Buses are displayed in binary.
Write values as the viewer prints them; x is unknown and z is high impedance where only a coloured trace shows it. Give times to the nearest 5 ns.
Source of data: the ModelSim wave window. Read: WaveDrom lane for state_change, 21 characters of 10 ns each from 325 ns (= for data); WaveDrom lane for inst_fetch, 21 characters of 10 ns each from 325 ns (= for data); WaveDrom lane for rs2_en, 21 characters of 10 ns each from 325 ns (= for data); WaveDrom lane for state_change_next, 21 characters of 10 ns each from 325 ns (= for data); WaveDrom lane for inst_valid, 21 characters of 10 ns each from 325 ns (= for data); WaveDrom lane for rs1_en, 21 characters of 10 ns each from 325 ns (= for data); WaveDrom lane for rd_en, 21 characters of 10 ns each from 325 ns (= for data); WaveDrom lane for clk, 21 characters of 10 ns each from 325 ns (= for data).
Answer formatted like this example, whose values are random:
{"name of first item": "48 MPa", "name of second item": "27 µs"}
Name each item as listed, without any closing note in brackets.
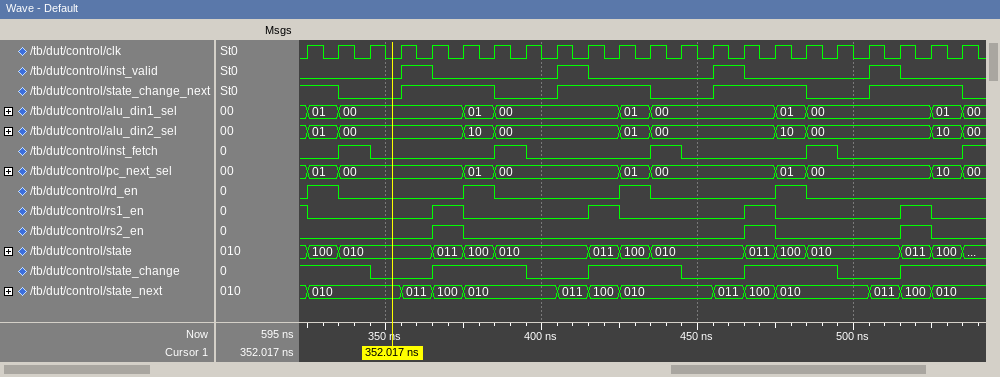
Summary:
{"WaveDrom lane for state_change, 21 characters of 10 ns each from 325 ns": "{name: 'state_change', wave: '1.0.1..0.1..0.1..0.1.'}", "WaveDrom lane for inst_fetch, 21 characters of 10 ns each from 325 ns": "{name: 'inst_fetch', wave: '010...10...10...10...'}", "WaveDrom lane for rs2_en, 21 characters of 10 ns each from 325 ns": "{name: 'rs2_en', wave: '0...10........10...10'}", "WaveDrom lane for state_change_next, 21 characters of 10 ns each from 325 ns": "{name: 'state_change_next', wave: '10.1..0.1..0.1..0.1..'}", "WaveDrom lane for inst_valid, 21 characters of 10 ns each from 325 ns": "{name: 'inst_valid', wave: '0..10...10...10...10.'}", "WaveDrom lane for rs1_en, 21 characters of 10 ns each from 325 ns": "{name: 'rs1_en', wave: '0...10...10...10...10'}", "WaveDrom lane for rd_en, 21 characters of 10 ns each from 325 ns": "{name: 'rd_en', wave: '10...10...10...10....'}", "WaveDrom lane for clk, 21 characters of 10 ns each from 325 ns": "{name: 'clk', wave: 'p....................'}"}
